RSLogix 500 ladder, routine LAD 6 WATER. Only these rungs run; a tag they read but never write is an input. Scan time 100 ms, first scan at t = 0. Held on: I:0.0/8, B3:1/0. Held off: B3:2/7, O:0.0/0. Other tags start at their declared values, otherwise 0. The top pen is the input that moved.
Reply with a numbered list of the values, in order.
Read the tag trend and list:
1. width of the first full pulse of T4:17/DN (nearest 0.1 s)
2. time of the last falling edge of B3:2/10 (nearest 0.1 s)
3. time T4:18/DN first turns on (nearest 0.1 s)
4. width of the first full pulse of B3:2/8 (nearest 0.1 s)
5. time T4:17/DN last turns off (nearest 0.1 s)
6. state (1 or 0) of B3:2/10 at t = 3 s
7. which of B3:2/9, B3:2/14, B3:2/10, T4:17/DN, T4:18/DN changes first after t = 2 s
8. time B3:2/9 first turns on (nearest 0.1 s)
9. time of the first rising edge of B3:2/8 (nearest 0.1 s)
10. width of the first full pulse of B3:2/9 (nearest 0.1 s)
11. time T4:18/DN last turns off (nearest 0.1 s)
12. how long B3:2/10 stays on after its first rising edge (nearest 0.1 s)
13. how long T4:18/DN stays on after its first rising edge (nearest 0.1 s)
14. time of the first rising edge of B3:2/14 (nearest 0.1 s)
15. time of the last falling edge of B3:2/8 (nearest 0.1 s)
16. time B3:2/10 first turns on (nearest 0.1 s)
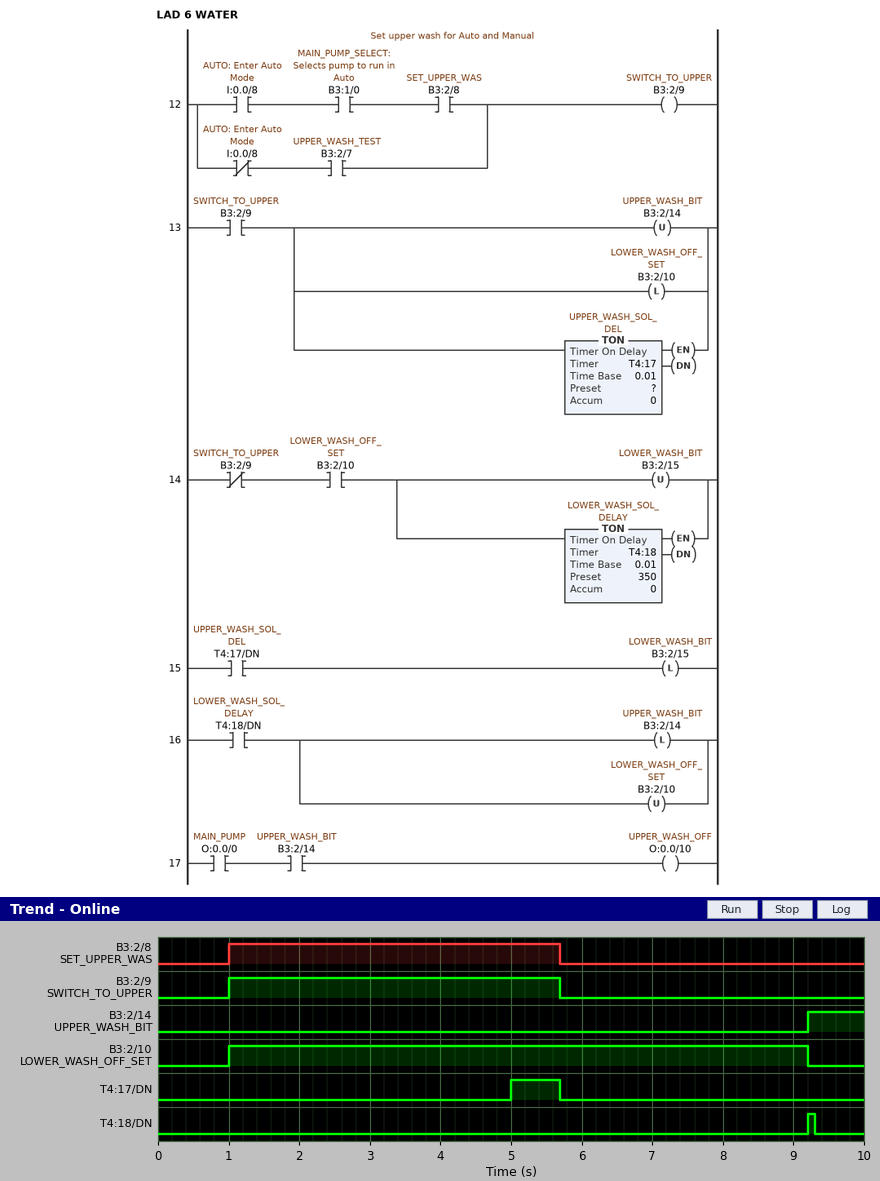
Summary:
1. 0.7 s
2. 9.2 s
3. 9.2 s
4. 4.7 s
5. 5.7 s
6. 1
7. T4:17/DN
8. 1.0 s
9. 1.0 s
10. 4.7 s
11. 9.3 s
12. 8.2 s
13. 0.1 s
14. 9.2 s
15. 5.7 s
16. 1.0 s
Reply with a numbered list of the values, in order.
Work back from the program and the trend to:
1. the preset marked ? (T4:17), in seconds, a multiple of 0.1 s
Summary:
1. 4.0 s
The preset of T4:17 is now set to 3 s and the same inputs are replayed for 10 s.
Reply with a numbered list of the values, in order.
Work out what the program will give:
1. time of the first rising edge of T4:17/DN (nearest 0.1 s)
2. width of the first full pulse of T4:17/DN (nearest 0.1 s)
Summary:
1. 4.0 s
2. 1.7 s
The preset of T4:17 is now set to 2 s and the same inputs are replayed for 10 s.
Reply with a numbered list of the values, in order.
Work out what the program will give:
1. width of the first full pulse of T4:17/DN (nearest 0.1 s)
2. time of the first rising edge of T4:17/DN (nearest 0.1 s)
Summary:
1. 2.7 s
2. 3.0 s
